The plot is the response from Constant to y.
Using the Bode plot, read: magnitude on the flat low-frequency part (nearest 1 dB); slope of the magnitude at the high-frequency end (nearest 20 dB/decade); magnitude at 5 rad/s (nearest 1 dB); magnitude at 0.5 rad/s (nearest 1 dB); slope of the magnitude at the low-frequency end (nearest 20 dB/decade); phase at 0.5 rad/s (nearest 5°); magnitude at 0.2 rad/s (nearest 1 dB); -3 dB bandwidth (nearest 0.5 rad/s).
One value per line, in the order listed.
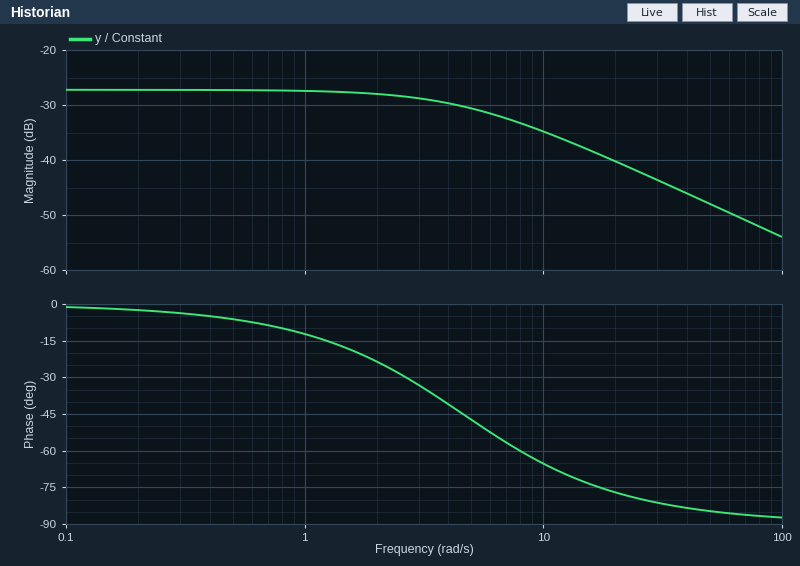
-27 dB
-20 dB/decade
-31 dB
-27 dB
0 dB/decade
-5°
-27 dB
4.5 rad/s
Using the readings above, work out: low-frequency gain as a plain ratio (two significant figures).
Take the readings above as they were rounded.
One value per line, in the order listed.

0.045
